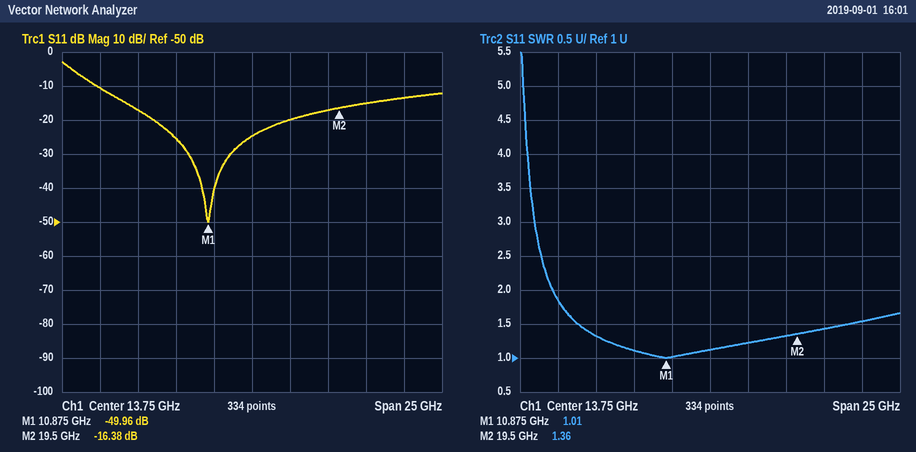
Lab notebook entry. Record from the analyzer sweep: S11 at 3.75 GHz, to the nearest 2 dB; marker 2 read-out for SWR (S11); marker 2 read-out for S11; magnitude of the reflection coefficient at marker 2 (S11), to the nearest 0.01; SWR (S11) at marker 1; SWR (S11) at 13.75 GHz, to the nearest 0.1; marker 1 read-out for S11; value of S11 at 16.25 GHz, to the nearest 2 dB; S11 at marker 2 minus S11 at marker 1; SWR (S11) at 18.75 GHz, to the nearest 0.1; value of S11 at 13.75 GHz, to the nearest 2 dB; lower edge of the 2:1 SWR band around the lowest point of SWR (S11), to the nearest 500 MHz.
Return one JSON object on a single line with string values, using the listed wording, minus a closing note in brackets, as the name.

{"S11 at 3.75 GHz, to the nearest 2 dB": "-10 dB", "marker 2 read-out for SWR": "1.36", "marker 2 read-out for S11": "-16.38 dB", "magnitude of the reflection coefficient at marker 2 (S11), to the nearest 0.01": "0.15", "SWR (S11) at marker 1": "1.01", "SWR (S11) at 13.75 GHz, to the nearest 0.1": "1.1", "marker 1 read-out for S11": "-49.96 dB", "value of S11 at 16.25 GHz, to the nearest 2 dB": "-20 dB", "S11 at marker 2 minus S11 at marker 1": "33.58 dB", "SWR (S11) at 18.75 GHz, to the nearest 0.1": "1.3", "value of S11 at 13.75 GHz, to the nearest 2 dB": "-24 dB", "lower edge of the 2:1 SWR band around the lowest point of SWR (S11), to the nearest 500 MHz": "3.5 GHz"}
